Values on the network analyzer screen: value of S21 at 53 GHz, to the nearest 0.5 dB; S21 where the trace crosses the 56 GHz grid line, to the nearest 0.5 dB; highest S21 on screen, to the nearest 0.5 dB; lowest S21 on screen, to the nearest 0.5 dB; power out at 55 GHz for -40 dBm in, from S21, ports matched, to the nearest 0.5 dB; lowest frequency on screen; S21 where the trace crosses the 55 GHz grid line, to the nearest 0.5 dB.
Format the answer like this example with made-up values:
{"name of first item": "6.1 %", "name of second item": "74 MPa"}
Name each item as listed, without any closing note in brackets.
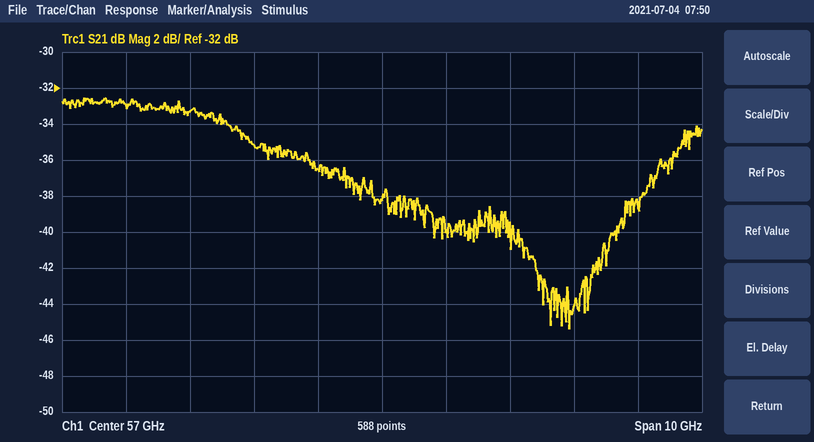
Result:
{"value of S21 at 53 GHz, to the nearest 0.5 dB": "-33.0 dB", "S21 where the trace crosses the 56 GHz grid line, to the nearest 0.5 dB": "-36.5 dB", "highest S21 on screen, to the nearest 0.5 dB": "-32.5 dB", "lowest S21 on screen, to the nearest 0.5 dB": "-45.5 dB", "power out at 55 GHz for -40 dBm in, from S21, ports matched, to the nearest 0.5 dB": "-75.0 dBm", "lowest frequency on screen": "52 GHz", "S21 where the trace crosses the 55 GHz grid line, to the nearest 0.5 dB": "-35.0 dB"}
